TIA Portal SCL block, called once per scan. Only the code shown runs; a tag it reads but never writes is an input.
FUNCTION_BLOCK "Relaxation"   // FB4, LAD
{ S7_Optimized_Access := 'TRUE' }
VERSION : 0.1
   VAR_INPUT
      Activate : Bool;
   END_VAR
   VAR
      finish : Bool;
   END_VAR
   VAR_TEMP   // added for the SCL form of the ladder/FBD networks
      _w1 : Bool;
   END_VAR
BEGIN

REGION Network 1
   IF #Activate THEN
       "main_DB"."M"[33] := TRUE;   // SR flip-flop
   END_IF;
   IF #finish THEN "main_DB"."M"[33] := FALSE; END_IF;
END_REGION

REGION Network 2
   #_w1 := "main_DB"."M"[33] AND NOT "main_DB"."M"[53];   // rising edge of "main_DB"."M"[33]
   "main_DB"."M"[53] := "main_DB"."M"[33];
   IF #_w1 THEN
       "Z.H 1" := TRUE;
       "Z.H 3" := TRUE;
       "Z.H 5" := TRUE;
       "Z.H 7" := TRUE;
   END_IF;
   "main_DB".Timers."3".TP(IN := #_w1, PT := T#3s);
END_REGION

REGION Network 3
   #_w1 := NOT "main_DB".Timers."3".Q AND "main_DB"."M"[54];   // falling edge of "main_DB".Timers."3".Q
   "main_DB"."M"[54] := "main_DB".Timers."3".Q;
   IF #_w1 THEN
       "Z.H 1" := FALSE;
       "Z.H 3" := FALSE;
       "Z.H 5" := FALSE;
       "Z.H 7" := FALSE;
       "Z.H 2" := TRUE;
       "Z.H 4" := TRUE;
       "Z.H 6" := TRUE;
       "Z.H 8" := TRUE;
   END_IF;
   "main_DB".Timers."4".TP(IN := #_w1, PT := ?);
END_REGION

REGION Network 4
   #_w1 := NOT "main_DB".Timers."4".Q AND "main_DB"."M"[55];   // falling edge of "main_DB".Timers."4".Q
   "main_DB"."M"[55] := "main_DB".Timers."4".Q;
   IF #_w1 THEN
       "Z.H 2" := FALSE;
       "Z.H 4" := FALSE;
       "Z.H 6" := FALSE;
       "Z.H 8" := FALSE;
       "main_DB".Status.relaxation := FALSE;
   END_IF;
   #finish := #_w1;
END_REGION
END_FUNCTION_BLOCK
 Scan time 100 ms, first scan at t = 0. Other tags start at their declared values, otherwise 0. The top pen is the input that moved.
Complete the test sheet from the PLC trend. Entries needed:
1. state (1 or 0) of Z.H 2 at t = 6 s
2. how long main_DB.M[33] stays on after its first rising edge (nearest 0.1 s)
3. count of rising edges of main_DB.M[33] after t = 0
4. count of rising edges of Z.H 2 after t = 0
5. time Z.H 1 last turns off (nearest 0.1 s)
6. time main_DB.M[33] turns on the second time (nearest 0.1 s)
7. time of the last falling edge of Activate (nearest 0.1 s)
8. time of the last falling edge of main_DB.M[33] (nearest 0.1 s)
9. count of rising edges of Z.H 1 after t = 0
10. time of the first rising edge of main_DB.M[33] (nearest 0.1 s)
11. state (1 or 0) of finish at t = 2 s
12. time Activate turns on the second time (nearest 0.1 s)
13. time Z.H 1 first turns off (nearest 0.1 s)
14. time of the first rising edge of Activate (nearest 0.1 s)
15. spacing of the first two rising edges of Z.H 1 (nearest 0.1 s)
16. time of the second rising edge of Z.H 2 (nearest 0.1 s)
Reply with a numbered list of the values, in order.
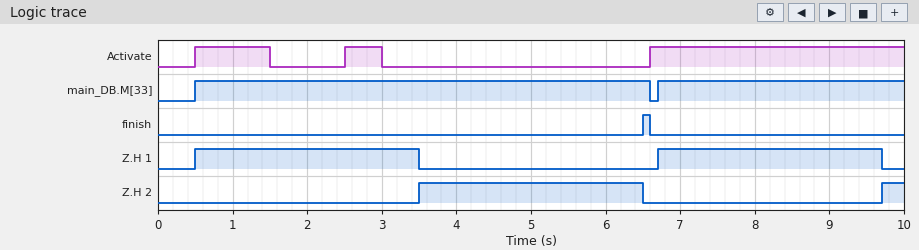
1. 1
2. 6.1 s
3. 2
4. 2
5. 9.7 s
6. 6.7 s
7. 3.0 s
8. 6.6 s
9. 2
10. 0.5 s
11. 0
12. 2.5 s
13. 3.5 s
14. 0.5 s
15. 6.2 s
16. 9.7 s
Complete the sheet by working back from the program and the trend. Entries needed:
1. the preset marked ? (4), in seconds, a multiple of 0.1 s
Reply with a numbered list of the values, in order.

1. 3.0 s
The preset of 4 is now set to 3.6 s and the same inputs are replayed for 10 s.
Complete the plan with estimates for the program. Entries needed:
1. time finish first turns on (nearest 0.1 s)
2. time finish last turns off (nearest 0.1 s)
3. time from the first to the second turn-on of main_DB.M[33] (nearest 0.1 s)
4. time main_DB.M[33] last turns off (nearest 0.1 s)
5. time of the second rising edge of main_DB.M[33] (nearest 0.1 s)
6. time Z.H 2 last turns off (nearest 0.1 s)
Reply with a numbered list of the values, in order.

1. 7.1 s
2. 7.2 s
3. 6.8 s
4. 7.2 s
5. 7.3 s
6. 7.1 s
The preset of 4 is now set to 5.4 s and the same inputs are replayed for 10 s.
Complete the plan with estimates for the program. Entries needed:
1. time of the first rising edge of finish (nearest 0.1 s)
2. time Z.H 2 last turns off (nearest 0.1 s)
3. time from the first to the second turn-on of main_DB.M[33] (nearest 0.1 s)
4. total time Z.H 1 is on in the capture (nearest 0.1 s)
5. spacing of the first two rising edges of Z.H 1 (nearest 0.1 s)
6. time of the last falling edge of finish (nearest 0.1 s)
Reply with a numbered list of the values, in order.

1. 8.9 s
2. 8.9 s
3. 8.6 s
4. 3.9 s
5. 8.6 s
6. 9.0 s
